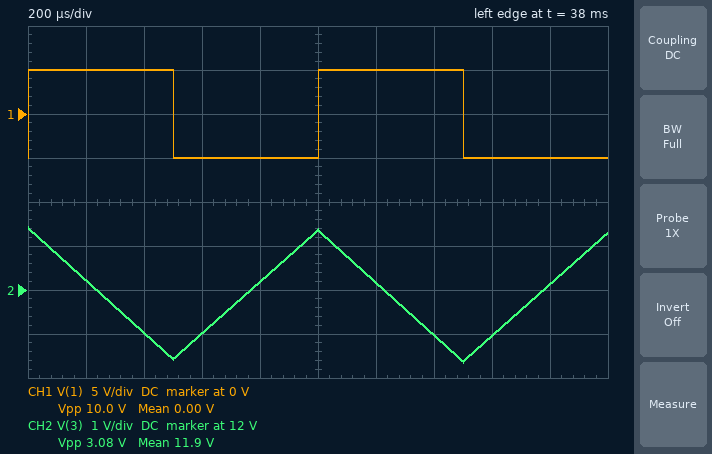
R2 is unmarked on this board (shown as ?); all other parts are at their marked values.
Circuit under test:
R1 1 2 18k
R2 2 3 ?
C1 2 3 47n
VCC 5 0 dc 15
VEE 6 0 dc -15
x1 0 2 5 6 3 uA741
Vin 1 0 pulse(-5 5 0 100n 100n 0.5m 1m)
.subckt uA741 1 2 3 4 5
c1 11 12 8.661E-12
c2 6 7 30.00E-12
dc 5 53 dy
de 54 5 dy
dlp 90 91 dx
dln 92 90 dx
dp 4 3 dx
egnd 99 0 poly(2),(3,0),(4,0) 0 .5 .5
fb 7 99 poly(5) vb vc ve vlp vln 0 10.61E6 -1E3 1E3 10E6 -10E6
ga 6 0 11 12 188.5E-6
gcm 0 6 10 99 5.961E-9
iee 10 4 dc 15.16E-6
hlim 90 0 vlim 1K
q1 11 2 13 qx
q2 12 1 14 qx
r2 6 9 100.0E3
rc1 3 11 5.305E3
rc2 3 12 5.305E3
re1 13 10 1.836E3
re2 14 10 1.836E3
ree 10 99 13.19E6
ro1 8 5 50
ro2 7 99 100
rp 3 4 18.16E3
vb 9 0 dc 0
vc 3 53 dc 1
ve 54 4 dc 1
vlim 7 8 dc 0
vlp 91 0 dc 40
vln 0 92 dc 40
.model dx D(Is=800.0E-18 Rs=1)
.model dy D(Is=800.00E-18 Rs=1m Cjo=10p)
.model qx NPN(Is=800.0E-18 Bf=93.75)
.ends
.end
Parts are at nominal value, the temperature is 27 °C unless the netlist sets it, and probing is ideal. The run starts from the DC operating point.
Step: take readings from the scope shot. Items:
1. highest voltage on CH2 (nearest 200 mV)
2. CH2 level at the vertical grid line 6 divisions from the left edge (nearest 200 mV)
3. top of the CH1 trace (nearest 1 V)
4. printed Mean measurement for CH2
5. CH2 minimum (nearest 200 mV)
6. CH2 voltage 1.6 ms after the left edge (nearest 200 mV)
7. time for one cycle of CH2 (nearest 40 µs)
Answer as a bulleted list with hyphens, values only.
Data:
- 13.4 V
- 12.2 V
- 5 V
- 11.9 V
- 10.4 V
- 11.0 V
- 1.00 ms
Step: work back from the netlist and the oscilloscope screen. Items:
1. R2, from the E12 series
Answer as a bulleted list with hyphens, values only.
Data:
- 4.7 MΩ
